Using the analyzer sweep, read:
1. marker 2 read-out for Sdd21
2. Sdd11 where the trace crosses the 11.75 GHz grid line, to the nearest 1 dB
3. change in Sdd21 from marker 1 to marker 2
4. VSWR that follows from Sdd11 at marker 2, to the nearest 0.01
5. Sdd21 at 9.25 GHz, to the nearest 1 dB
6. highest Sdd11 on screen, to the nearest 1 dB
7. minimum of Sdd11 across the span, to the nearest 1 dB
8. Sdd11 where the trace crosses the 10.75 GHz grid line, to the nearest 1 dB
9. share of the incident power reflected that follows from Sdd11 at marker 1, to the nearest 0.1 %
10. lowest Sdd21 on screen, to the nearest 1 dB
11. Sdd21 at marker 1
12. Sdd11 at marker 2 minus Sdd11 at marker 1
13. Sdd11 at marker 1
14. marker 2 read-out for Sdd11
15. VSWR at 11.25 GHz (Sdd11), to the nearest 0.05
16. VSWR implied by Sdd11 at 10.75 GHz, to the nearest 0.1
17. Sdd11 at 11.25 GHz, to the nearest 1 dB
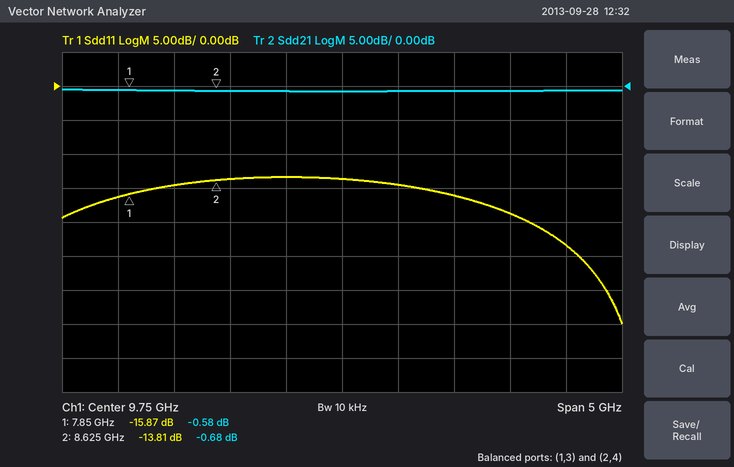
-0.68 dB
-23 dB
-0.10 dB
1.51
-1 dB
-13 dB
-35 dB
-16 dB
2.6 %
-1 dB
-0.58 dB
2.06 dB
-15.87 dB
-13.81 dB
1.25
1.4
-19 dB
